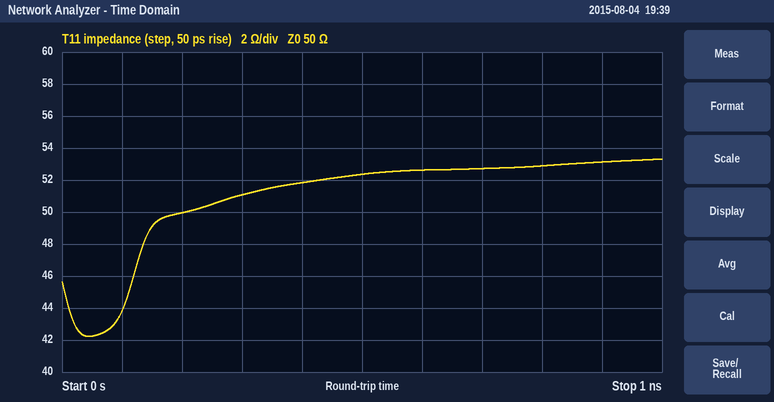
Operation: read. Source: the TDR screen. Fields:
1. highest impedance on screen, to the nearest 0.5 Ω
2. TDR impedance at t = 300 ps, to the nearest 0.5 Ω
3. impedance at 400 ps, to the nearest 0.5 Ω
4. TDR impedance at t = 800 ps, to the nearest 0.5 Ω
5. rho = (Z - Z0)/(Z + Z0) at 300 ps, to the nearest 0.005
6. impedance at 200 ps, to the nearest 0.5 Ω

53.5 Ω
51.0 Ω
52.0 Ω
53.0 Ω
+0.010
50.0 Ω
